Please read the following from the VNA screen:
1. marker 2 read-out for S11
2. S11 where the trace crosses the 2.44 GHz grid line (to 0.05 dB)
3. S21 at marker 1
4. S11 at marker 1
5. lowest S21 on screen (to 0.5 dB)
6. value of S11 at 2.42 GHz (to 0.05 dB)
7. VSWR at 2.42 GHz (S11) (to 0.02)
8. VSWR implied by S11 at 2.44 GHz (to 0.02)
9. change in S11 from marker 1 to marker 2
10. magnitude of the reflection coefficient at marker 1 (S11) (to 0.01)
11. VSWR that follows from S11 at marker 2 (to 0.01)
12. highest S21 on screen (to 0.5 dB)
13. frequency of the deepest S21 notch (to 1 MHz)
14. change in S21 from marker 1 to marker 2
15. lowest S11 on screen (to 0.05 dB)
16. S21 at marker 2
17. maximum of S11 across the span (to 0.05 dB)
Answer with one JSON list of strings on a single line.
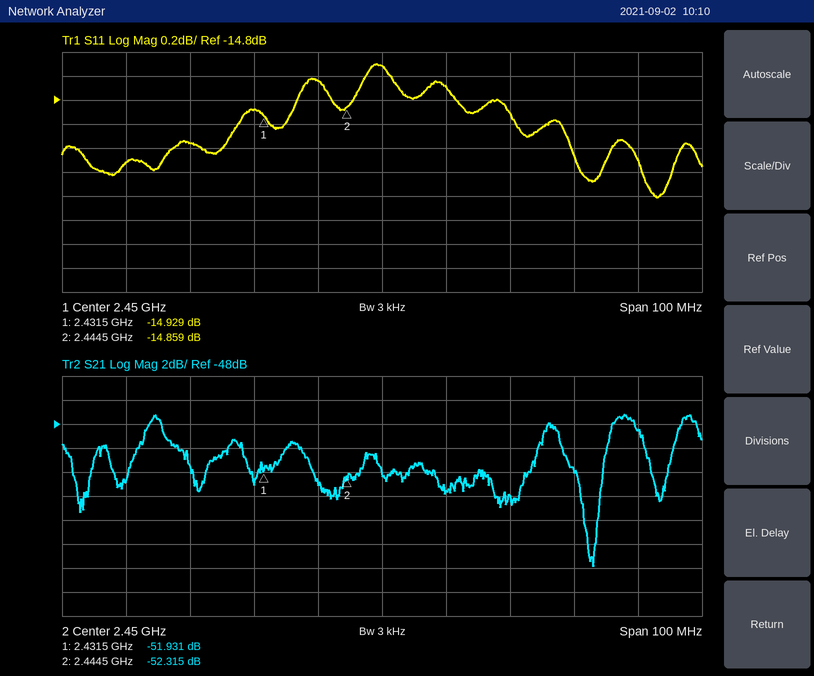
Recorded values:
["-14.859 dB", "-14.65 dB", "-51.931 dB", "-14.929 dB", "-60.0 dB", "-15.15 dB", "1.42", "1.46", "0.070 dB", "0.18", "1.44", "-47.0 dB", "2.483 GHz", "-0.384 dB", "-15.60 dB", "-52.315 dB", "-14.50 dB"]
